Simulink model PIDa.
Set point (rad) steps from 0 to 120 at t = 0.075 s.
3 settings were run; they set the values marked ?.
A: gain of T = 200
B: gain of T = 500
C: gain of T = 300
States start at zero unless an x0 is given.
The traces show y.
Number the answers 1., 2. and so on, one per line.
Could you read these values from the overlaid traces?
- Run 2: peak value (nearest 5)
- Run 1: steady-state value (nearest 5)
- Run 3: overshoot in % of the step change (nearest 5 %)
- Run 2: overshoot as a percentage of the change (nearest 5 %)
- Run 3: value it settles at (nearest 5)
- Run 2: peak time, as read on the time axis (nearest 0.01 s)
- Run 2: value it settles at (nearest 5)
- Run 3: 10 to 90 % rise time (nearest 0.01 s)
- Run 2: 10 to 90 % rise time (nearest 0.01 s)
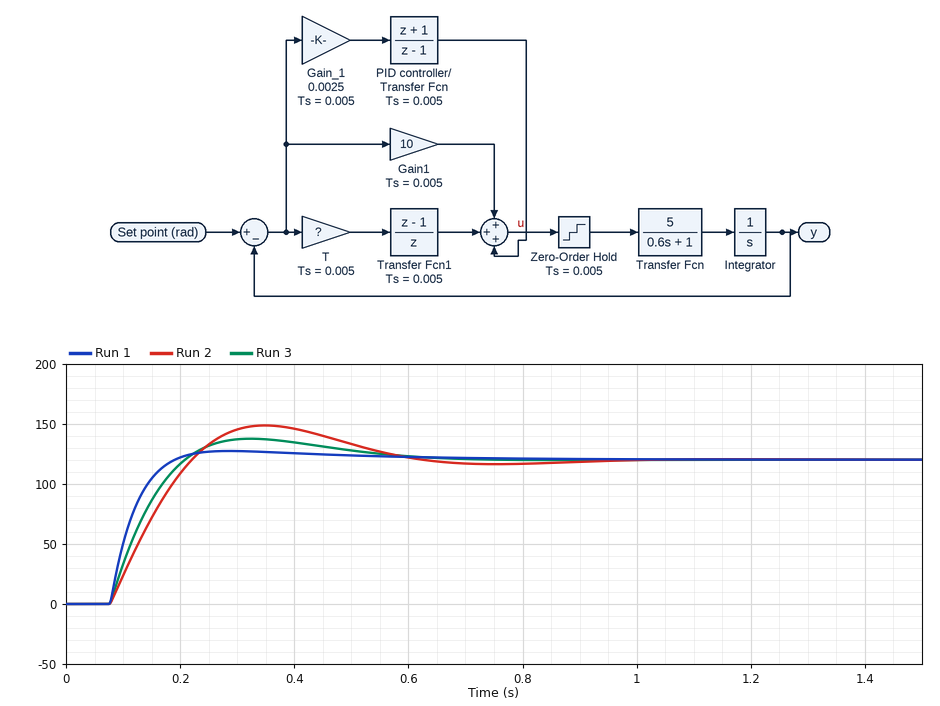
1. 150
2. 120
3. 15 %
4. 25 %
5. 120
6. 0.35 s
7. 120
8. 0.10 s
9. 0.11 s
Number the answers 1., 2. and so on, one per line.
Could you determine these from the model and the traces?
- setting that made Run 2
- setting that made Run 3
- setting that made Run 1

1. A
2. C
3. B
